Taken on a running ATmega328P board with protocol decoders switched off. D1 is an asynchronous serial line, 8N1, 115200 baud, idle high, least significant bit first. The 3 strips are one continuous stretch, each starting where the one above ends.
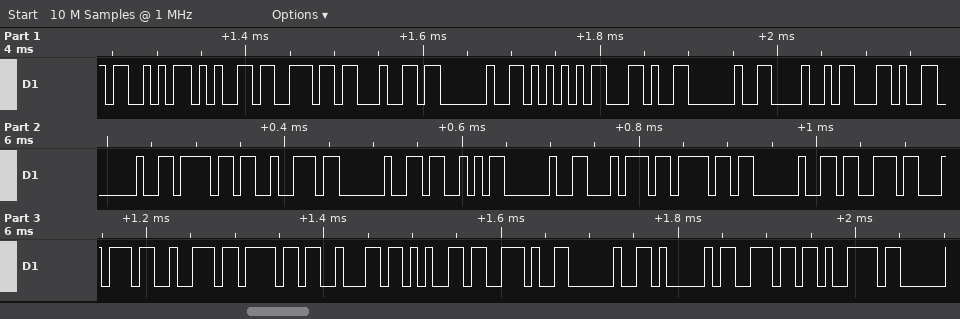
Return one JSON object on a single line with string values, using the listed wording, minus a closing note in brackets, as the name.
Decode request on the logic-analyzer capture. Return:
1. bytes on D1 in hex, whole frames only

{"bytes on D1 in hex, whole frames only": "53 65 6E 64 20 55 2C 20 48 2C 20 6F 72 20 53 20 74 6F 20 73 74 72 6F 62 65 2E 20 41 6E 79"}
